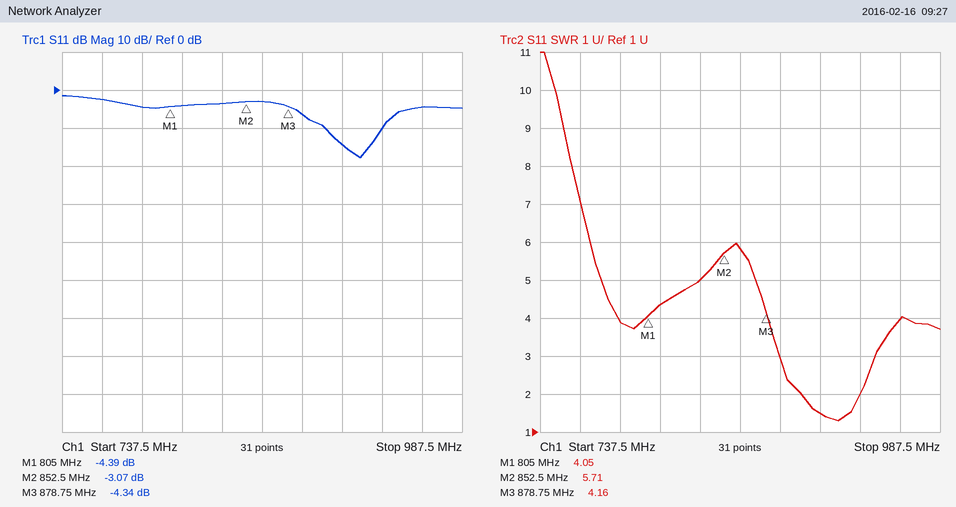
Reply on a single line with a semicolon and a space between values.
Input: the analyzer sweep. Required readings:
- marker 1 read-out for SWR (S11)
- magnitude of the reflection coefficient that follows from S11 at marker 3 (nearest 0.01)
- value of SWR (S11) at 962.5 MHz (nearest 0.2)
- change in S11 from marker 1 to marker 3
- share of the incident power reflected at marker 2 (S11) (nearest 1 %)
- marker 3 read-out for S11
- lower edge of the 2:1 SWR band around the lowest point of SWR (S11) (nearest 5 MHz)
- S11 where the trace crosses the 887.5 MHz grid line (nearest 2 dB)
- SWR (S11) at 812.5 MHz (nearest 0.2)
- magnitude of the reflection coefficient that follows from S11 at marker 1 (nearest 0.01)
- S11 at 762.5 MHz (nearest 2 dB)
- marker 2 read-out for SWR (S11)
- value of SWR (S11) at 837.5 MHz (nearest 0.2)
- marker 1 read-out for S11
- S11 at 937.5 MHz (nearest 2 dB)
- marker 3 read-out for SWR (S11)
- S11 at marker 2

4.05; 0.61; 4.0; 0.05 dB; 49 %; -4.34 dB; 900 MHz; -6 dB; 4.4; 0.60; -2 dB; 5.71; 5.0; -4.39 dB; -10 dB; 4.16; -3.07 dB
